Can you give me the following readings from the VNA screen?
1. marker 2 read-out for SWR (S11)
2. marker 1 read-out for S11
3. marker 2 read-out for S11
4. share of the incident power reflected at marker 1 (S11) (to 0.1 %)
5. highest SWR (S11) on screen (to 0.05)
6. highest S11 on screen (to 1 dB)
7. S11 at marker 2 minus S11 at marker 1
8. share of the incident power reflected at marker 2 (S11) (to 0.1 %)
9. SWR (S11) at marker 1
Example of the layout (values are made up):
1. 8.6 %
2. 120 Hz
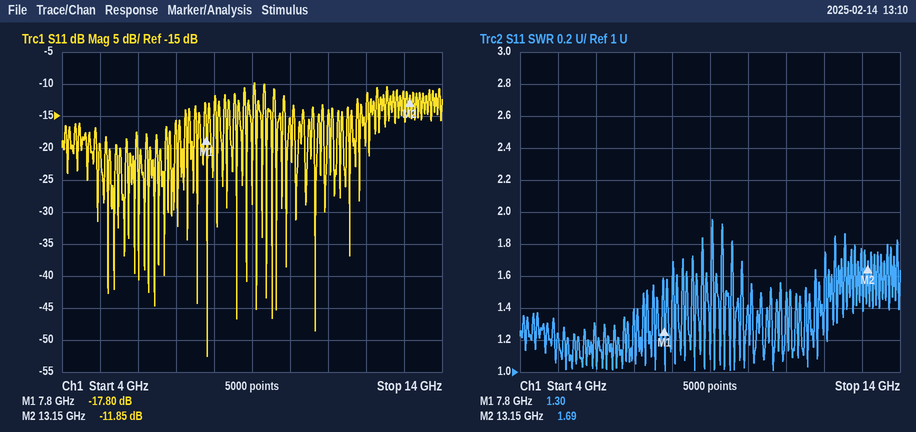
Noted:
1. 1.69
2. -17.80 dB
3. -11.85 dB
4. 1.7 %
5. 1.95
6. -10 dB
7. 5.95 dB
8. 6.5 %
9. 1.30
